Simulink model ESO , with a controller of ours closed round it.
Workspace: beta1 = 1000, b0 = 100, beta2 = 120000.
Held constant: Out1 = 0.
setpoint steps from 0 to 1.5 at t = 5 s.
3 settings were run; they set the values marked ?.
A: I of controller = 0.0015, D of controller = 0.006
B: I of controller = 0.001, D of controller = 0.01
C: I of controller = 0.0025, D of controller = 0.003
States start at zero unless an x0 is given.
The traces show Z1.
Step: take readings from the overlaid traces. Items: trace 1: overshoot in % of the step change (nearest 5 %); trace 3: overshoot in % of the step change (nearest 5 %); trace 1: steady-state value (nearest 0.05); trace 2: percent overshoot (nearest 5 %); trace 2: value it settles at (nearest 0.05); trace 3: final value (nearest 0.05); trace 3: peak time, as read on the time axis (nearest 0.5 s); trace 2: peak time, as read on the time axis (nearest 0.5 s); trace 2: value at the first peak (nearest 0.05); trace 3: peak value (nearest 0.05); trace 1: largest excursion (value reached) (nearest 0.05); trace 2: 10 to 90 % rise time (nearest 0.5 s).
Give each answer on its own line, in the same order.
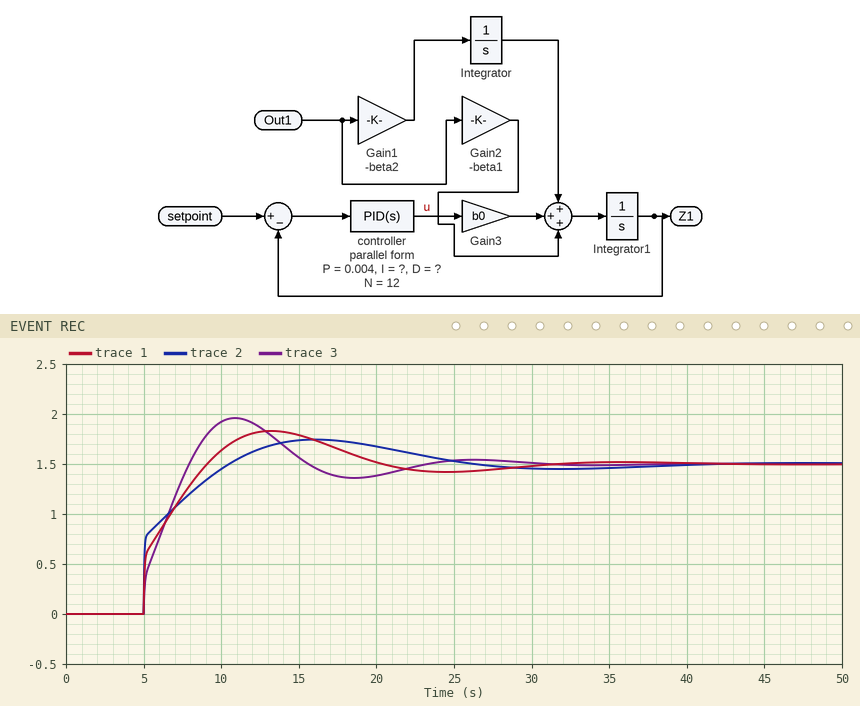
20 %
30 %
1.50
15 %
1.50
1.50
11.0 s
16.0 s
1.75
1.95
1.85
4.0 s
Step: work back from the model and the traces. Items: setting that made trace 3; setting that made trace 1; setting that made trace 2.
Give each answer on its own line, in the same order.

C
A
B
